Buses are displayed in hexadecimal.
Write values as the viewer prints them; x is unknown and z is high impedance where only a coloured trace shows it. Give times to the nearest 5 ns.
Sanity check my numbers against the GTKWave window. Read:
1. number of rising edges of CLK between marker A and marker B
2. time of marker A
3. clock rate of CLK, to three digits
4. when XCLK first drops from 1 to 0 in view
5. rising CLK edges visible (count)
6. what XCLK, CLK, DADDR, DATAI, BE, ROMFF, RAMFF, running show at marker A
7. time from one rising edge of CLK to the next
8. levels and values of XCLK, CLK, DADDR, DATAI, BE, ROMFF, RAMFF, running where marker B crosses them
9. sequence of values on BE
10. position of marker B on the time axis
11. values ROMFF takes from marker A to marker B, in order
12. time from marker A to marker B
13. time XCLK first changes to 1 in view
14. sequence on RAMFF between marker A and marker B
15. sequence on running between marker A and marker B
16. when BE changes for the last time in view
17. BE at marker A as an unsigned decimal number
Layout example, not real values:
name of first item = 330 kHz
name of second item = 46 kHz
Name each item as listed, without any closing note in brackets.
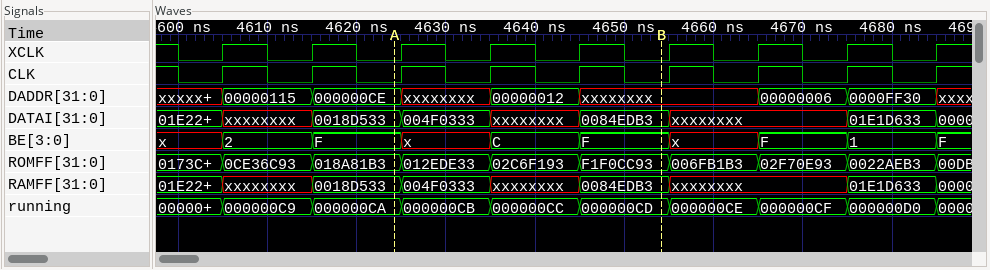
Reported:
number of rising edges of CLK between marker A and marker B = 3
time of marker A = 4625 ns
clock rate of CLK, to three digits = 100 MHz
when XCLK first drops from 1 to 0 in view = 4600 ns
rising CLK edges visible = 9
what XCLK, CLK, DADDR, DATAI, BE, ROMFF, RAMFF, running show at marker A = XCLK=0, CLK=0, DADDR=000000CE, DATAI=0018D533, BE=F, ROMFF=018A81B3, RAMFF=0018D533, running=000000CA
time from one rising edge of CLK to the next = 10 ns
levels and values of XCLK, CLK, DADDR, DATAI, BE, ROMFF, RAMFF, running where marker B crosses them = XCLK=0, CLK=0, DADDR=xxxxxxxx, DATAI=0084EDB3, BE=F, ROMFF=F1F0CC93, RAMFF=0084EDB3, running=000000CD
sequence of values on BE = x, 2, F, x, C, F, x, F, 1, F
position of marker B on the time axis = 4655 ns
values ROMFF takes from marker A to marker B, in order = 018A81B3, 012EDE33, 02C6F193, F1F0CC93
time from marker A to marker B = 30 ns
time XCLK first changes to 1 in view = 4605 ns
sequence on RAMFF between marker A and marker B = 0018D533, 004F0333, xxxxxxxx, 0084EDB3
sequence on running between marker A and marker B = 000000CA, 000000CB, 000000CC, 000000CD
when BE changes for the last time in view = 4685 ns
BE at marker A as an unsigned decimal number = 15
